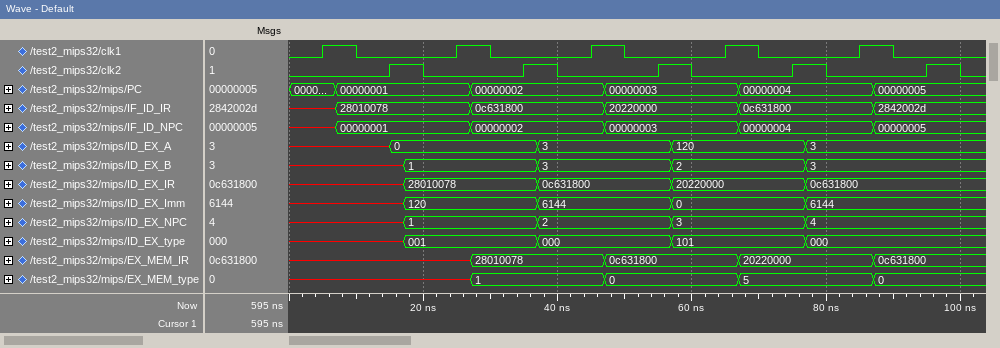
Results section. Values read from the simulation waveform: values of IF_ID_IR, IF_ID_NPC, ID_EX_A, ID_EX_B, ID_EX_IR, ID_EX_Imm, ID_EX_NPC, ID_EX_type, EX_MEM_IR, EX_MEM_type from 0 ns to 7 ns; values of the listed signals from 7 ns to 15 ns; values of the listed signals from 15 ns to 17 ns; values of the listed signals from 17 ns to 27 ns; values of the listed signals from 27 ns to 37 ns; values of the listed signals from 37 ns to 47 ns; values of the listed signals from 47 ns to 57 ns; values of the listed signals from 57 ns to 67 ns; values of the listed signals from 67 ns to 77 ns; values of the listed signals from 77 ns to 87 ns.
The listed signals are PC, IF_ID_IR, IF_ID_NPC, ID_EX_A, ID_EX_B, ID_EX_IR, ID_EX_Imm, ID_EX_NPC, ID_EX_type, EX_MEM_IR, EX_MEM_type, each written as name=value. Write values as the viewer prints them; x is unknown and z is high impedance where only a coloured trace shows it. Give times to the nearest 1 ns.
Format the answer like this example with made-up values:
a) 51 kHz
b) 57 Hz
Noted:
a) IF_ID_IR=x, IF_ID_NPC=x, ID_EX_A=x, ID_EX_B=x, ID_EX_IR=x, ID_EX_Imm=x, ID_EX_NPC=x, ID_EX_type=x, EX_MEM_IR=x, EX_MEM_type=x
b) PC=00000001, IF_ID_IR=28010078, IF_ID_NPC=00000001, ID_EX_A=x, ID_EX_B=x, ID_EX_IR=x, ID_EX_Imm=x, ID_EX_NPC=x, ID_EX_type=x, EX_MEM_IR=x, EX_MEM_type=x
c) PC=00000001, IF_ID_IR=28010078, IF_ID_NPC=00000001, ID_EX_A=0, ID_EX_B=x, ID_EX_IR=x, ID_EX_Imm=x, ID_EX_NPC=x, ID_EX_type=x, EX_MEM_IR=x, EX_MEM_type=x
d) PC=00000001, IF_ID_IR=28010078, IF_ID_NPC=00000001, ID_EX_A=0, ID_EX_B=1, ID_EX_IR=28010078, ID_EX_Imm=120, ID_EX_NPC=1, ID_EX_type=001, EX_MEM_IR=x, EX_MEM_type=x
e) PC=00000002, IF_ID_IR=0c631800, IF_ID_NPC=00000002, ID_EX_A=0, ID_EX_B=1, ID_EX_IR=28010078, ID_EX_Imm=120, ID_EX_NPC=1, ID_EX_type=001, EX_MEM_IR=28010078, EX_MEM_type=1
f) PC=00000002, IF_ID_IR=0c631800, IF_ID_NPC=00000002, ID_EX_A=3, ID_EX_B=3, ID_EX_IR=0c631800, ID_EX_Imm=6144, ID_EX_NPC=2, ID_EX_type=000, EX_MEM_IR=28010078, EX_MEM_type=1
g) PC=00000003, IF_ID_IR=20220000, IF_ID_NPC=00000003, ID_EX_A=3, ID_EX_B=3, ID_EX_IR=0c631800, ID_EX_Imm=6144, ID_EX_NPC=2, ID_EX_type=000, EX_MEM_IR=0c631800, EX_MEM_type=0
h) PC=00000003, IF_ID_IR=20220000, IF_ID_NPC=00000003, ID_EX_A=120, ID_EX_B=2, ID_EX_IR=20220000, ID_EX_Imm=0, ID_EX_NPC=3, ID_EX_type=101, EX_MEM_IR=0c631800, EX_MEM_type=0
i) PC=00000004, IF_ID_IR=0c631800, IF_ID_NPC=00000004, ID_EX_A=120, ID_EX_B=2, ID_EX_IR=20220000, ID_EX_Imm=0, ID_EX_NPC=3, ID_EX_type=101, EX_MEM_IR=20220000, EX_MEM_type=5
j) PC=00000004, IF_ID_IR=0c631800, IF_ID_NPC=00000004, ID_EX_A=3, ID_EX_B=3, ID_EX_IR=0c631800, ID_EX_Imm=6144, ID_EX_NPC=4, ID_EX_type=000, EX_MEM_IR=20220000, EX_MEM_type=5
